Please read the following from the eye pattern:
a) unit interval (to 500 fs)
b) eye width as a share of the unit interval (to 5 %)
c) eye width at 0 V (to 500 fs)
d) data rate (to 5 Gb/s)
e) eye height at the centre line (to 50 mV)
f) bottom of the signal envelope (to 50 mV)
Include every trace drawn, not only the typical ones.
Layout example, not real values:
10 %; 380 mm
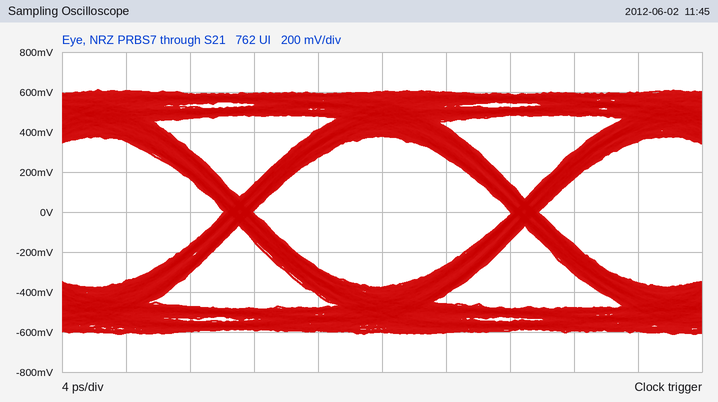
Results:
18.0 ps; 90 %; 16.0 ps; 55 Gb/s; 750 mV; -600 mV
